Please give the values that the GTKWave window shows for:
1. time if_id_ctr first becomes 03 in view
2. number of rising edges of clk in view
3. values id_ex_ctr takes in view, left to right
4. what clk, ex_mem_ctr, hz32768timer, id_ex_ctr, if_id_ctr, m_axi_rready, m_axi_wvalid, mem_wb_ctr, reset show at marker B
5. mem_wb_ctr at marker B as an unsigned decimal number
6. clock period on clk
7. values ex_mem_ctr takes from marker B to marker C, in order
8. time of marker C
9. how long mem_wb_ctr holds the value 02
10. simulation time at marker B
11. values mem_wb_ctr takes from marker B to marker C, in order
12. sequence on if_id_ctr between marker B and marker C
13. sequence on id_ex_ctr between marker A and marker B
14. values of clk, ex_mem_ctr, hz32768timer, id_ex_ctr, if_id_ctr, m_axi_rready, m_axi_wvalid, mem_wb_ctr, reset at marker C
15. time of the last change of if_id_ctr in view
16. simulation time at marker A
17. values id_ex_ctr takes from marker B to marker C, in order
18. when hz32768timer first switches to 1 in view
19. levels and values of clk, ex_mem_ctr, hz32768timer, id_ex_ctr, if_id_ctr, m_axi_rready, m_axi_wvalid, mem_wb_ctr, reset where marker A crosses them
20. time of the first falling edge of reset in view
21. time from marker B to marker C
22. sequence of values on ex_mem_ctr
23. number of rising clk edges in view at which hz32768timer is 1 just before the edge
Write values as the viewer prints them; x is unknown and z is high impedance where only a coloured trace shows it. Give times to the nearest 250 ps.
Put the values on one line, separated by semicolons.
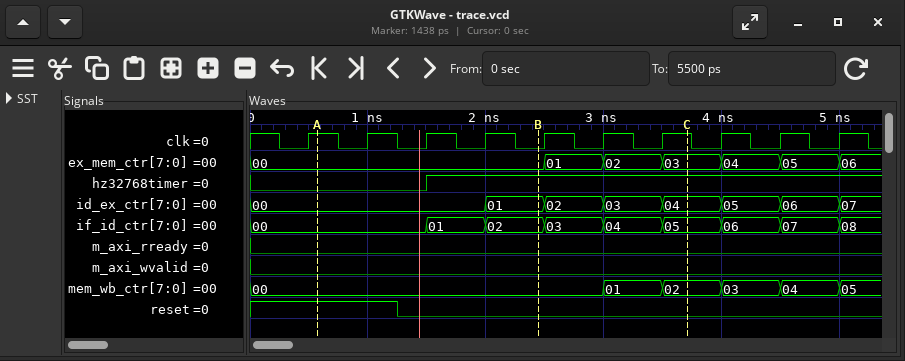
2500 ps; 10; 00, 01, 02, 03, 04, 05, 06, 07; clk=0, ex_mem_ctr=00, hz32768timer=1, id_ex_ctr=01, if_id_ctr=02, m_axi_rready=0, m_axi_wvalid=0, mem_wb_ctr=00, reset=0; 0; 500 ps; 00, 01, 02, 03; 3750 ps; 500 ps; 2500 ps; 00, 01, 02; 02, 03, 04, 05; 00, 01; clk=1, ex_mem_ctr=03, hz32768timer=1, id_ex_ctr=04, if_id_ctr=05, m_axi_rready=0, m_axi_wvalid=0, mem_wb_ctr=02, reset=0; 5000 ps; 500 ps; 01, 02, 03, 04; 1500 ps; clk=1, ex_mem_ctr=00, hz32768timer=0, id_ex_ctr=00, if_id_ctr=00, m_axi_rready=0, m_axi_wvalid=0, mem_wb_ctr=00, reset=1; 1250 ps; 1250 ps; 00, 01, 02, 03, 04, 05, 06; 7
